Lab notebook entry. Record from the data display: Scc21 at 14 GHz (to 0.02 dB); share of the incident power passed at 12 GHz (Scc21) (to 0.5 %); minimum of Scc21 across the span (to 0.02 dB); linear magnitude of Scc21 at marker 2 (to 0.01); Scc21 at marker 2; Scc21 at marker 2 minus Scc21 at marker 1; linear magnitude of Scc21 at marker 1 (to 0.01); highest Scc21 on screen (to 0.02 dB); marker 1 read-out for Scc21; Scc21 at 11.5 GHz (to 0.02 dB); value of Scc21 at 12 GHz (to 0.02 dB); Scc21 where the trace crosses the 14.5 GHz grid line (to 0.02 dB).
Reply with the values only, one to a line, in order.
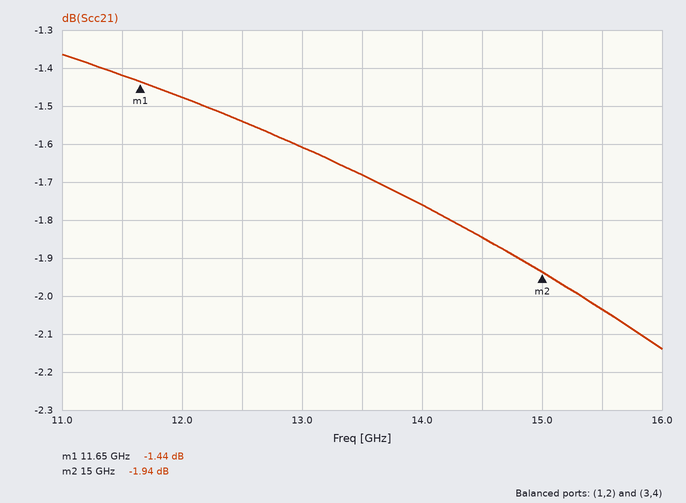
-1.76 dB
71.0 %
-2.14 dB
0.80
-1.94 dB
-0.50 dB
0.85
-1.36 dB
-1.44 dB
-1.42 dB
-1.48 dB
-1.84 dB
